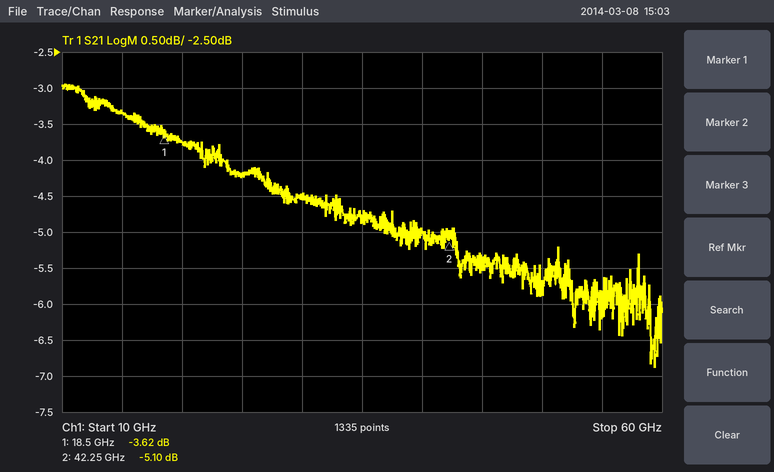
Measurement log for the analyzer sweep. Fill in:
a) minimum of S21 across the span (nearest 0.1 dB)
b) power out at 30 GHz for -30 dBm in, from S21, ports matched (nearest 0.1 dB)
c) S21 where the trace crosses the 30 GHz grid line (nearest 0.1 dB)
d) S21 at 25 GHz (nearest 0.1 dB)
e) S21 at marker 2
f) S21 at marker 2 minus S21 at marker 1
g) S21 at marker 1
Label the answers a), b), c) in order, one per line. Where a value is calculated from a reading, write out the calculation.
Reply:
a) -6.9 dB
b) -30 dBm + (-4.5 dB) = -34.5 dBm
c) -4.5 dB
d) -4.2 dB
e) -5.10 dB
f) -5.1 − (-3.62) = -1.48 dB
g) -3.62 dB
